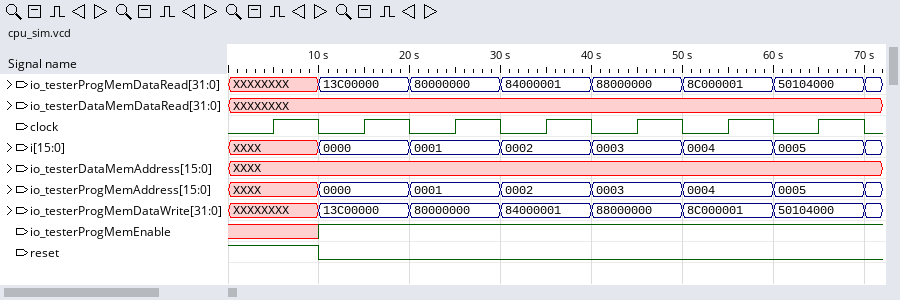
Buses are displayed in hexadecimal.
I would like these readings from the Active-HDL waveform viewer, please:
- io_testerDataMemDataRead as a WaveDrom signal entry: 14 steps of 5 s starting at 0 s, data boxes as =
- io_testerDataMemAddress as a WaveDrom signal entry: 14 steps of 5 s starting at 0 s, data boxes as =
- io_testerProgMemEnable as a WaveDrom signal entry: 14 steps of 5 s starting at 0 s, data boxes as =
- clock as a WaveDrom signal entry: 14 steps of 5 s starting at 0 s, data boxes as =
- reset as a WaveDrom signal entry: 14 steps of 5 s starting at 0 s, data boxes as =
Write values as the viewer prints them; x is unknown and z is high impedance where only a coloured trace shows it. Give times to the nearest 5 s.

{name: 'io_testerDataMemDataRead', wave: 'x.............'}
{name: 'io_testerDataMemAddress', wave: 'x.............'}
{name: 'io_testerProgMemEnable', wave: 'x.1...........'}
{name: 'clock', wave: '01010101010101'}
{name: 'reset', wave: '1.0...........'}
